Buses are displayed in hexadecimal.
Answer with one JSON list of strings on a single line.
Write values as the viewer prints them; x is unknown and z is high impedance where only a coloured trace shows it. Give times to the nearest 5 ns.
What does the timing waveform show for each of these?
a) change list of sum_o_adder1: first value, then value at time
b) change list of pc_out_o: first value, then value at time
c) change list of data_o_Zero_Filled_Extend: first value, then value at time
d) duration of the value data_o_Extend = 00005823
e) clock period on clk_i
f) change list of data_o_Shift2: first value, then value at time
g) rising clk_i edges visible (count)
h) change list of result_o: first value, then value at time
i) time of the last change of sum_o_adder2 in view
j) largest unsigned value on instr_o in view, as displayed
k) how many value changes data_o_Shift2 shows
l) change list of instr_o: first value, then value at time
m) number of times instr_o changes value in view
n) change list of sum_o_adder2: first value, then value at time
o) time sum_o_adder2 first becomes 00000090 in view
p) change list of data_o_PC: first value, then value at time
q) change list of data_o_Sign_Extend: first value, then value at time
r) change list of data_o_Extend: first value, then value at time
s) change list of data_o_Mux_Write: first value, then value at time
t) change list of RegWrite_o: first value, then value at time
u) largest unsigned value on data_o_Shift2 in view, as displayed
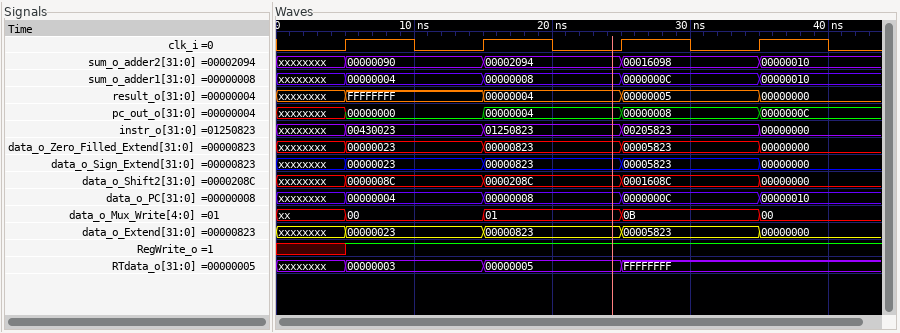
["xxxxxxxx, 00000004 at 5 ns, 00000008 at 15 ns, 0000000C at 25 ns, 00000010 at 35 ns", "xxxxxxxx, 00000000 at 5 ns, 00000004 at 15 ns, 00000008 at 25 ns, 0000000C at 35 ns", "xxxxxxxx, 00000023 at 5 ns, 00000823 at 15 ns, 00005823 at 25 ns, 00000000 at 35 ns", "10 ns", "10 ns", "xxxxxxxx, 0000008C at 5 ns, 0000208C at 15 ns, 0001608C at 25 ns, 00000000 at 35 ns", "4", "xxxxxxxx, FFFFFFFF at 5 ns, 00000004 at 15 ns, 00000005 at 25 ns, 00000000 at 35 ns", "35 ns", "01250823", "4", "xxxxxxxx, 00430023 at 5 ns, 01250823 at 15 ns, 00205823 at 25 ns, 00000000 at 35 ns", "4", "xxxxxxxx, 00000090 at 5 ns, 00002094 at 15 ns, 00016098 at 25 ns, 00000010 at 35 ns", "5 ns", "xxxxxxxx, 00000004 at 5 ns, 00000008 at 15 ns, 0000000C at 25 ns, 00000010 at 35 ns", "xxxxxxxx, 00000023 at 5 ns, 00000823 at 15 ns, 00005823 at 25 ns, 00000000 at 35 ns", "xxxxxxxx, 00000023 at 5 ns, 00000823 at 15 ns, 00005823 at 25 ns, 00000000 at 35 ns", "xx, 00 at 5 ns, 01 at 15 ns, 0B at 25 ns, 00 at 35 ns", "x, 1 at 5 ns", "0001608C"]
